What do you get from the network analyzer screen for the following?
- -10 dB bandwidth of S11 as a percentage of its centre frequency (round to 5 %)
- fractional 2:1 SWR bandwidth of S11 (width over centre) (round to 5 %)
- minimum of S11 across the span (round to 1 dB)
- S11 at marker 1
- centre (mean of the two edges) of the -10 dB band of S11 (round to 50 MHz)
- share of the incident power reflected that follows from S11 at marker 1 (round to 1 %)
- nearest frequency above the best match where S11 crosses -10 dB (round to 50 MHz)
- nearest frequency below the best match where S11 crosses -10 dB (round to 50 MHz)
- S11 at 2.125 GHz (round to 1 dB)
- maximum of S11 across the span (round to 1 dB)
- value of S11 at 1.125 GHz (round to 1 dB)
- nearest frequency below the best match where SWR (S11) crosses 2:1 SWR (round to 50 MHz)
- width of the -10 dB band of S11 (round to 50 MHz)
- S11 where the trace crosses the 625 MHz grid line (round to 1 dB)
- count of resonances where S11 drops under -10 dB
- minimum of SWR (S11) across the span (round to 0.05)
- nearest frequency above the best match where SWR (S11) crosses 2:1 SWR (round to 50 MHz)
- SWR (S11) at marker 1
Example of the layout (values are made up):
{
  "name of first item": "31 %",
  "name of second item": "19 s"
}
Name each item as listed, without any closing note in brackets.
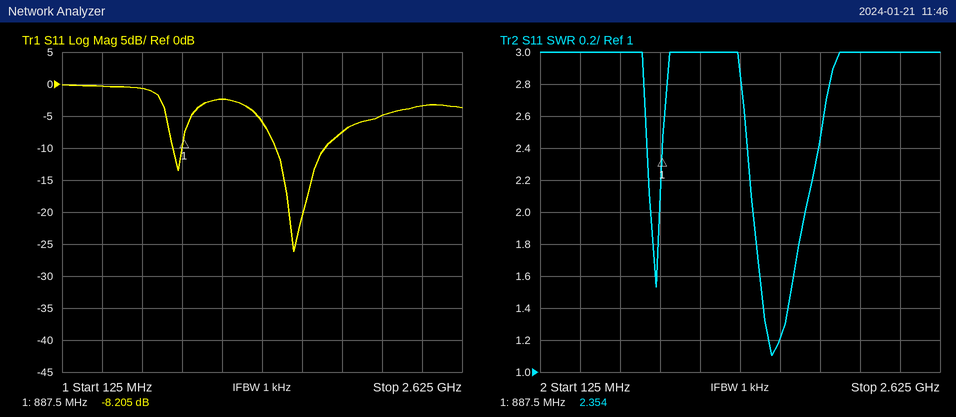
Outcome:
{
  "-10 dB bandwidth of S11 as a percentage of its centre frequency": "20 %",
  "fractional 2:1 SWR bandwidth of S11 (width over centre)": "20 %",
  "minimum of S11 across the span": "-26 dB",
  "S11 at marker 1": "-8.205 dB",
  "centre (mean of the two edges) of the -10 dB band of S11": "1.60 GHz",
  "share of the incident power reflected that follows from S11 at marker 1": "15 %",
  "nearest frequency above the best match where S11 crosses -10 dB": "1.75 GHz",
  "nearest frequency below the best match where S11 crosses -10 dB": "1.45 GHz",
  "S11 at 2.125 GHz": "-5 dB",
  "maximum of S11 across the span": "0 dB",
  "value of S11 at 1.125 GHz": "-2 dB",
  "nearest frequency below the best match where SWR (S11) crosses 2:1 SWR": "1.45 GHz",
  "width of the -10 dB band of S11": "300 MHz",
  "S11 where the trace crosses the 625 MHz grid line": "-1 dB",
  "count of resonances where S11 drops under -10 dB": "2",
  "minimum of SWR (S11) across the span": "1.10",
  "nearest frequency above the best match where SWR (S11) crosses 2:1 SWR": "1.80 GHz",
  "SWR (S11) at marker 1": "2.354"
}
